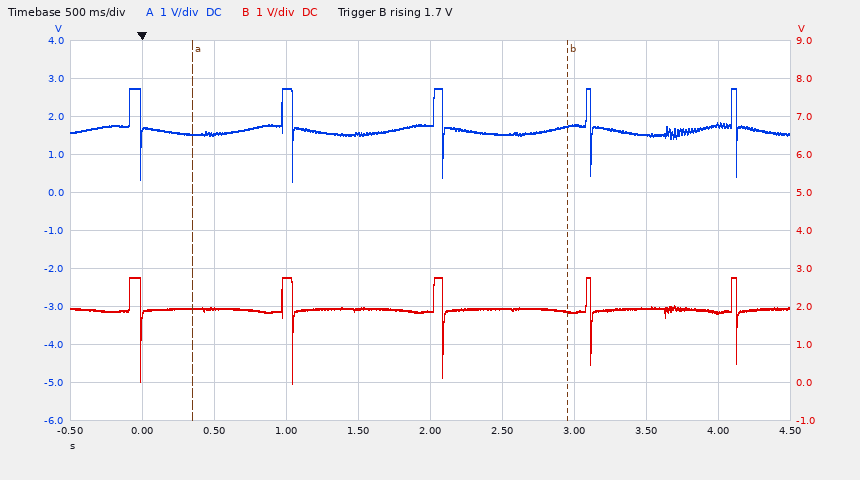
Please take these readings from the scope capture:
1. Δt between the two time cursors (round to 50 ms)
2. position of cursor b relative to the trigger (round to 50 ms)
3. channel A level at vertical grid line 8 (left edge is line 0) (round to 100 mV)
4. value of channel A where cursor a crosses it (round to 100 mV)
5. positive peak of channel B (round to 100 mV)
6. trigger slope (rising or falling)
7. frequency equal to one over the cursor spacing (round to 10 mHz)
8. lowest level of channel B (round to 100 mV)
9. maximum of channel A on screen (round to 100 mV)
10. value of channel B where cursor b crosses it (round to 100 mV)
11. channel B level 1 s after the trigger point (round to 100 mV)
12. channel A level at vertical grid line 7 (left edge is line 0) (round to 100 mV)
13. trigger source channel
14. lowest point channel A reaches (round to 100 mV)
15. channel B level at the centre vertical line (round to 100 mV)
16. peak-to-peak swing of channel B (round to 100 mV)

2.60 s
+2.95 s
1.5 V
1.5 V
2.8 V
rising
380 mHz
0.0 V
2.7 V
1.9 V
2.8 V
1.8 V
channel B
300 mV
1.9 V
2.8 V
